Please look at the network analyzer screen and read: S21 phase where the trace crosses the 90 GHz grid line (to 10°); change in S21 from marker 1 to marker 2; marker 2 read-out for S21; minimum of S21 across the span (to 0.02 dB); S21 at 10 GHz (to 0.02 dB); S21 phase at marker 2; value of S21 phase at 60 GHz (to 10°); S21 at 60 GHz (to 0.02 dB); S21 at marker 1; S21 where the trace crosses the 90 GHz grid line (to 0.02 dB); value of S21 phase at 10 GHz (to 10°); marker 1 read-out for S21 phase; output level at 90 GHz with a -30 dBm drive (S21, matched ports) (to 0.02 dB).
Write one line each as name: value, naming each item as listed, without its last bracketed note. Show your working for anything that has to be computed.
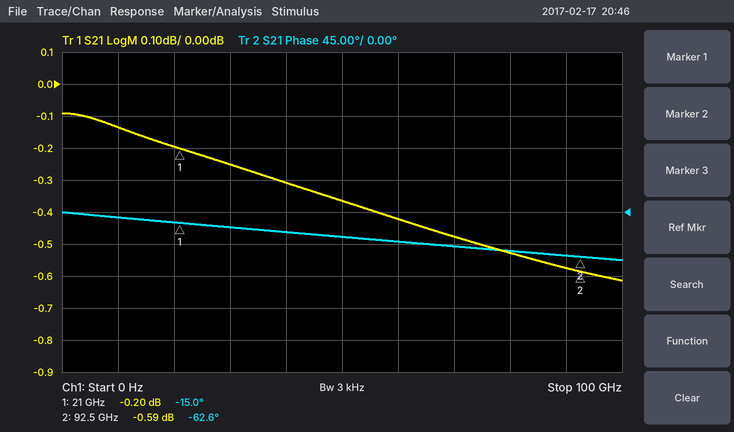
S21 phase where the trace crosses the 90 GHz grid line: -60°
change in S21 from marker 1 to marker 2: -0.59 − (-0.2) = -0.39 dB
marker 2 read-out for S21: -0.59 dB
minimum of S21 across the span: -0.62 dB
S21 at 10 GHz: -0.14 dB
S21 phase at marker 2: -62.6°
value of S21 phase at 60 GHz: -40°
S21 at 60 GHz: -0.42 dB
S21 at marker 1: -0.20 dB
S21 where the trace crosses the 90 GHz grid line: -0.58 dB
value of S21 phase at 10 GHz: -10°
marker 1 read-out for S21 phase: -15.0°
output level at 90 GHz with a -30 dBm drive (S21, matched ports): -30 dBm + (-0.58 dB) = -30.58 dBm
